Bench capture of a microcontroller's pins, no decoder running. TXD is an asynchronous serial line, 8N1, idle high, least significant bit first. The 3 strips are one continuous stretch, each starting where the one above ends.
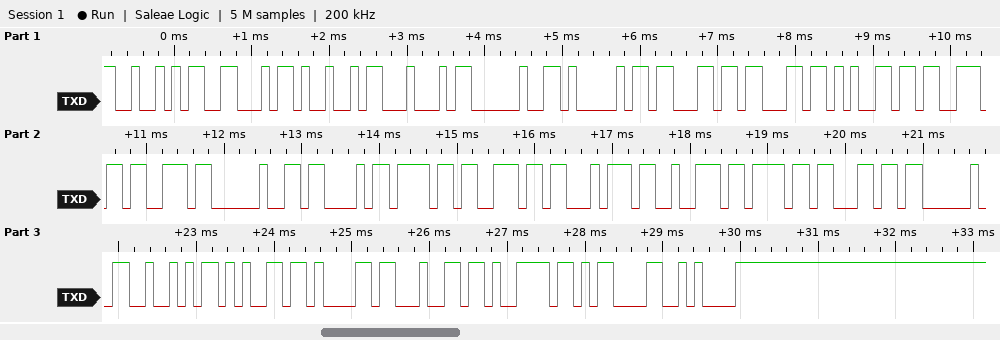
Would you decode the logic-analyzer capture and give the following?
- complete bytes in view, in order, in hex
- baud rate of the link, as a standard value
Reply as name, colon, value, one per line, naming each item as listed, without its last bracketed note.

complete bytes in view, in order, in hex: 52 46 49 44 20 41 63 63 65 73 73 20 43 6F 6E 74 72 6F 6C 20 52 65 61 64 79 0D 0A
baud rate of the link, as a standard value: 9600 baud
